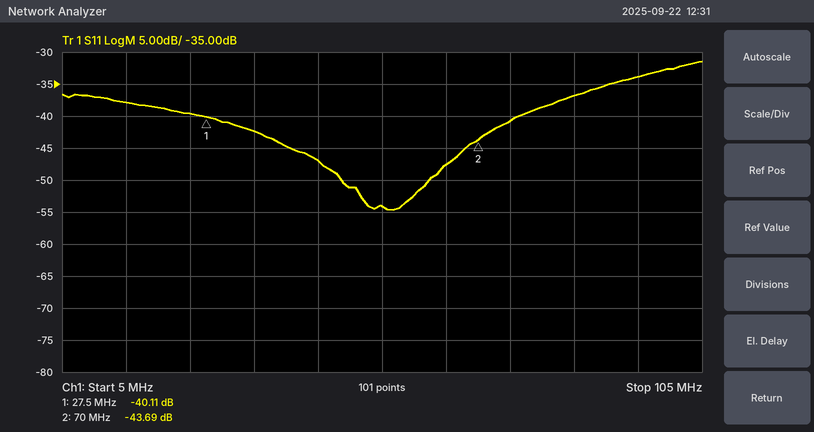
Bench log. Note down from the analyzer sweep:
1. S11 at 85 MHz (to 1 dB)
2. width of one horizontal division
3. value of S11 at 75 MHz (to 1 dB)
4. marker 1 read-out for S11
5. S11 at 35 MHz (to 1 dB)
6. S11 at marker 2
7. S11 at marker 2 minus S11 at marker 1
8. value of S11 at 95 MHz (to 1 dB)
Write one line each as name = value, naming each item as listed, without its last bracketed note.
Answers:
S11 at 85 MHz = -37 dB
width of one horizontal division = 10 MHz
value of S11 at 75 MHz = -41 dB
marker 1 read-out for S11 = -40.11 dB
S11 at 35 MHz = -42 dB
S11 at marker 2 = -43.69 dB
S11 at marker 2 minus S11 at marker 1 = -3.58 dB
value of S11 at 95 MHz = -34 dB
